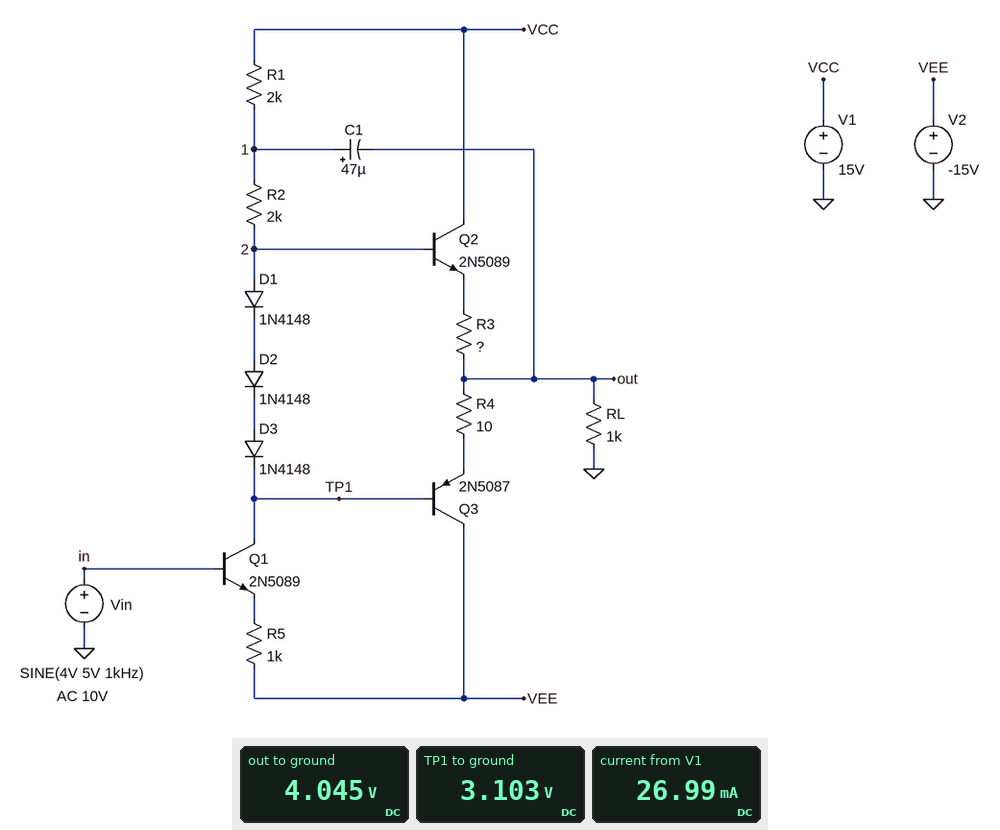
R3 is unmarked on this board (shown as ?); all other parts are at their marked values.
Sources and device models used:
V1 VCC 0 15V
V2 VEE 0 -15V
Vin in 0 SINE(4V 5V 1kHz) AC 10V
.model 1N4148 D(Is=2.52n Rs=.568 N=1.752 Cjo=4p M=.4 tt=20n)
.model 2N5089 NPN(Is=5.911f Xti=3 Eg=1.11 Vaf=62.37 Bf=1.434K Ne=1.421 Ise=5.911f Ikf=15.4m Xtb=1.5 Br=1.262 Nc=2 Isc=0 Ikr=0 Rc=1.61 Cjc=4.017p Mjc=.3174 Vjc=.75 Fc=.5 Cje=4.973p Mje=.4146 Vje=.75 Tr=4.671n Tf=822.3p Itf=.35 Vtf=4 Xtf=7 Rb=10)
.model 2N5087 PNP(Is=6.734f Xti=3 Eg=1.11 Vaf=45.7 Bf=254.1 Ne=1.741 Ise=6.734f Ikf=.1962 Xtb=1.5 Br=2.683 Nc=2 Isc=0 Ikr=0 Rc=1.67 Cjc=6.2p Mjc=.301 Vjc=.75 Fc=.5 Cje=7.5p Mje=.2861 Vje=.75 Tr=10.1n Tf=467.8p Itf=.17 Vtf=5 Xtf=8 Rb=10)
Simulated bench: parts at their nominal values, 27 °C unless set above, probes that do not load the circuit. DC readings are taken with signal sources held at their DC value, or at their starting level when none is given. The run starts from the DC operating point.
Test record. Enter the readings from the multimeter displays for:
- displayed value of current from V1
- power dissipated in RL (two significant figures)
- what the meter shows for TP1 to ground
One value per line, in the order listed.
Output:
26.99 mA
16 mW
3.103 V
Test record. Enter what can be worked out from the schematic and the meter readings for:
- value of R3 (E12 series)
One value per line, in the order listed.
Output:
6.8 Ω
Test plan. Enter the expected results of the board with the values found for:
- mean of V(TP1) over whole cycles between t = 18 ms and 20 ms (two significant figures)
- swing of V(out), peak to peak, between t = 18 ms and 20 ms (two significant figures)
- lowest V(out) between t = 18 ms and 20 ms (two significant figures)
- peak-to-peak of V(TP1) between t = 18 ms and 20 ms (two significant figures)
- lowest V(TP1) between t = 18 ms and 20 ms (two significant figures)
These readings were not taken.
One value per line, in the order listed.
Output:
3.1 V
9.8 V
-860 mV
9.9 V
-1.8 V
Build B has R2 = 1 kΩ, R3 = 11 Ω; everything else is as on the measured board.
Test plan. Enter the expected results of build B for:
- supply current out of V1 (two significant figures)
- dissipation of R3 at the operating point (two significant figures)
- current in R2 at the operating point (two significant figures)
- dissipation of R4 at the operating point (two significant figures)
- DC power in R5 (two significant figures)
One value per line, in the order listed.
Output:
25 mA
5.3 mW
3.3 mA
3.2 mW
330 mW
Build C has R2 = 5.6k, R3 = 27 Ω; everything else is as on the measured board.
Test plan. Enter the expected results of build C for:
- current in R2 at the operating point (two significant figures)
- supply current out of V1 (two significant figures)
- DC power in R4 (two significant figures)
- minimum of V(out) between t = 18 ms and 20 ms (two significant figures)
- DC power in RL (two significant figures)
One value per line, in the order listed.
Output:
1.3 mA
12 mA
440 µW
-1.0 V
15 mW
